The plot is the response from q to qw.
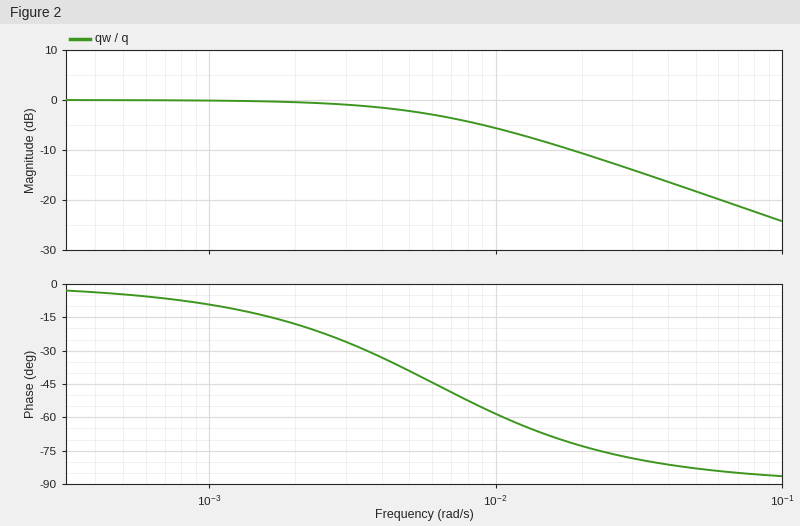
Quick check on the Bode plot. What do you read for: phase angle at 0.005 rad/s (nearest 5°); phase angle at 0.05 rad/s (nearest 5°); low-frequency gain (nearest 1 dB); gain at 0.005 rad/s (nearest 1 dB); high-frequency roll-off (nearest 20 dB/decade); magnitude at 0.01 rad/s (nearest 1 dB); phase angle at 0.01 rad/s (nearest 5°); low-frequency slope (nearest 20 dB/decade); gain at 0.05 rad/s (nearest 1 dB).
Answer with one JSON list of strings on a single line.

["-40°", "-85°", "0 dB", "-2 dB", "-20 dB/decade", "-6 dB", "-60°", "0 dB/decade", "-18 dB"]
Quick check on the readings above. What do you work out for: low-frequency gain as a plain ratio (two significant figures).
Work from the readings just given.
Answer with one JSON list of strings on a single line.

["1.0"]
